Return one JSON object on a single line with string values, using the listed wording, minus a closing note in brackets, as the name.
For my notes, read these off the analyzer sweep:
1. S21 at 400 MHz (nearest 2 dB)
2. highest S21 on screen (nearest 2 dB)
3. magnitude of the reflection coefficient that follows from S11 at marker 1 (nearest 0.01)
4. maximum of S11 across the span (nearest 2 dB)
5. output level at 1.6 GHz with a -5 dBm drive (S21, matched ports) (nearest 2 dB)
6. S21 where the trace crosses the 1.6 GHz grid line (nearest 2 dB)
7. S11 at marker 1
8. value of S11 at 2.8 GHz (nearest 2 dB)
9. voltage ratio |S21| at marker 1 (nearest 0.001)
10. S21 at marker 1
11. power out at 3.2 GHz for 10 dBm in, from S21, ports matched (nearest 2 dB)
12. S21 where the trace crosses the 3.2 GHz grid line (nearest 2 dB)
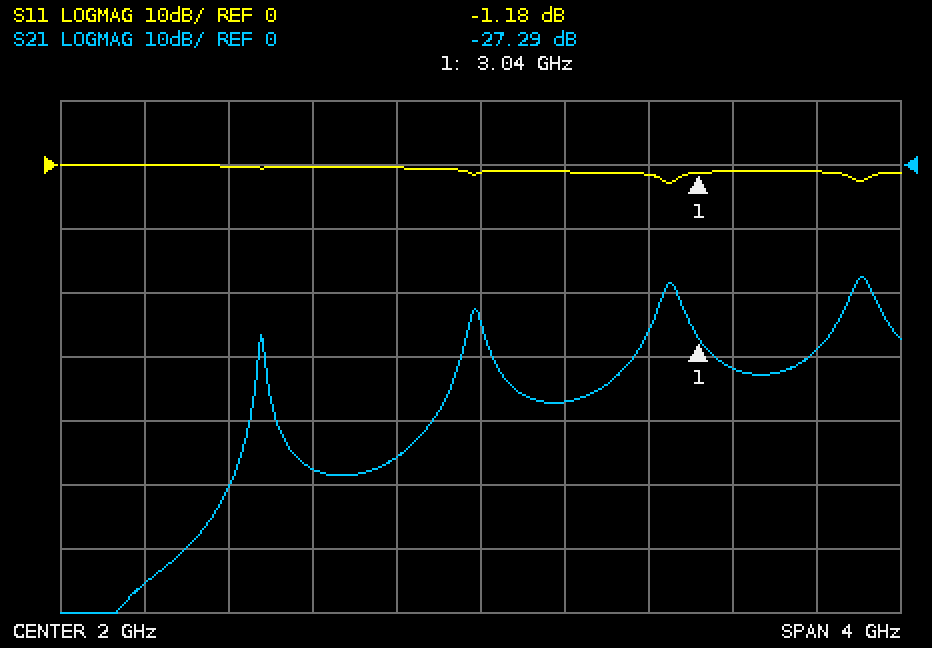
{"S21 at 400 MHz": "-66 dB", "highest S21 on screen": "-18 dB", "magnitude of the reflection coefficient that follows from S11 at marker 1": "0.87", "maximum of S11 across the span": "0 dB", "output level at 1.6 GHz with a -5 dBm drive (S21, matched ports)": "-50 dBm", "S21 where the trace crosses the 1.6 GHz grid line": "-46 dB", "S11 at marker 1": "-1.18 dB", "value of S11 at 2.8 GHz": "-2 dB", "voltage ratio |S21| at marker 1": "0.043", "S21 at marker 1": "-27.29 dB", "power out at 3.2 GHz for 10 dBm in, from S21, ports matched": "-22 dBm", "S21 where the trace crosses the 3.2 GHz grid line": "-32 dB"}
